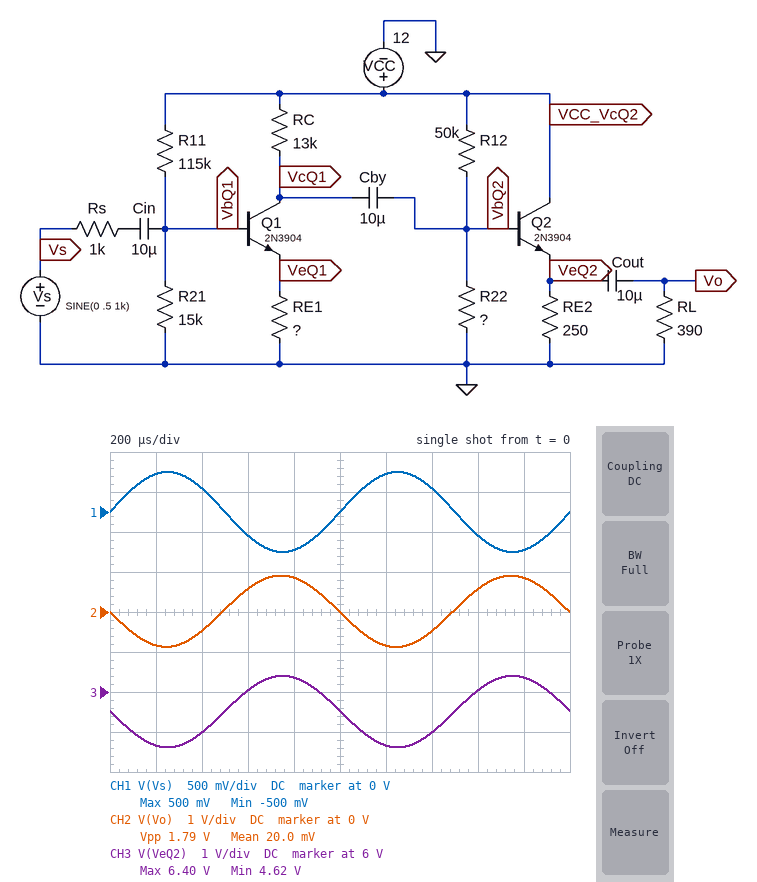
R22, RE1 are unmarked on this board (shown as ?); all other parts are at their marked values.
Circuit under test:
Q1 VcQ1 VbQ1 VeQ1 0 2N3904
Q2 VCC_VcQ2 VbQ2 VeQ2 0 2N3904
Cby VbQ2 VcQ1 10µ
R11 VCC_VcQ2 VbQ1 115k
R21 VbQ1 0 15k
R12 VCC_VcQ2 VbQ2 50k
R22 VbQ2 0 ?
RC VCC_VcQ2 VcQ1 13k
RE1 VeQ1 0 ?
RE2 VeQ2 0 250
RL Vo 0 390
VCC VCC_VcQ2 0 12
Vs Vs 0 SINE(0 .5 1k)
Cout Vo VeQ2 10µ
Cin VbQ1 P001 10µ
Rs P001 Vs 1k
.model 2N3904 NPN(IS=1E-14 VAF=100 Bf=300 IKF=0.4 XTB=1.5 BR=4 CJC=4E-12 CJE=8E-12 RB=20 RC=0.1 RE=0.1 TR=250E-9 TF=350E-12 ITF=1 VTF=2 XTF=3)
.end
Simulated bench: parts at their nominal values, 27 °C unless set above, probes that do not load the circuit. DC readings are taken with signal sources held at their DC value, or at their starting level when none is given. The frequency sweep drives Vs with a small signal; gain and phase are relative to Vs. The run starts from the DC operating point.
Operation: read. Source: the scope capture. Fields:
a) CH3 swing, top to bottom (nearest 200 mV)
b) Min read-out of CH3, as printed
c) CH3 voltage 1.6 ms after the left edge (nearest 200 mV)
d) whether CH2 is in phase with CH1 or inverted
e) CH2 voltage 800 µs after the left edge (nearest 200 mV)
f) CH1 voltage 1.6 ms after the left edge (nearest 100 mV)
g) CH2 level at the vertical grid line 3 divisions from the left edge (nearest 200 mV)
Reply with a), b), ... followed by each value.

a) 1.8 V
b) 4.62 V
c) 6.0 V
d) inverted
e) 800 mV
f) -300 mV
g) 600 mV
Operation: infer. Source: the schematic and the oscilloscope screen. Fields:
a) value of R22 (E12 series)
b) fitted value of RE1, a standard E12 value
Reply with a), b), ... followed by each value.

a) 150 kΩ
b) 3.9 kΩ
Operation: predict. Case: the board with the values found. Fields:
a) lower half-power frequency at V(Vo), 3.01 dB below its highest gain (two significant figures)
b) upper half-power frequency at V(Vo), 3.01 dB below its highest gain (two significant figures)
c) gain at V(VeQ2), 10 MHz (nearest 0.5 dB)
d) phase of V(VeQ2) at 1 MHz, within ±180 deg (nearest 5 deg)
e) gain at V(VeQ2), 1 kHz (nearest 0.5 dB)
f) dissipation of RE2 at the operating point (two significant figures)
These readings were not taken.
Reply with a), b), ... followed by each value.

a) 38 Hz
b) 3.1 MHz
c) -4.5 dB
d) 160 deg
e) 5.0 dB
f) 120 mW
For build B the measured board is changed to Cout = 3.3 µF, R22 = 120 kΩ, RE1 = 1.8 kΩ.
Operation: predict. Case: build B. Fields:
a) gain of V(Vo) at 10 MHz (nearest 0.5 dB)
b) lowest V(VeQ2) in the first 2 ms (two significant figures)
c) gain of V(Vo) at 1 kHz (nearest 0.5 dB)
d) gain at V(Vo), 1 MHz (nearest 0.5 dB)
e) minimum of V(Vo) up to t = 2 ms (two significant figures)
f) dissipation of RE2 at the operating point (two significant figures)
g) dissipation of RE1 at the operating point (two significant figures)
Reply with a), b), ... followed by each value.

a) 0.5 dB
b) 3.3 V
c) 11.5 dB
d) 11.0 dB
e) -1.8 V
f) 110 mW
g) 300 µW
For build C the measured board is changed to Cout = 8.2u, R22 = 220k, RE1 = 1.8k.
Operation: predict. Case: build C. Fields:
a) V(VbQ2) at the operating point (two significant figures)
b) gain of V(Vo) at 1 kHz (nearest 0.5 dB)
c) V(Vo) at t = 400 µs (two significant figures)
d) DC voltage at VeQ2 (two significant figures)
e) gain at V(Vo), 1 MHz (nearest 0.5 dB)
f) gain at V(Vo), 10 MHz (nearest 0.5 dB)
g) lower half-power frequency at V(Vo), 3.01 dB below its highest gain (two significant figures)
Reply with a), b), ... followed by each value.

a) 6.6 V
b) 12.0 dB
c) -1.0 V
d) 5.9 V
e) 11.5 dB
f) 0.5 dB
g) 46 Hz
